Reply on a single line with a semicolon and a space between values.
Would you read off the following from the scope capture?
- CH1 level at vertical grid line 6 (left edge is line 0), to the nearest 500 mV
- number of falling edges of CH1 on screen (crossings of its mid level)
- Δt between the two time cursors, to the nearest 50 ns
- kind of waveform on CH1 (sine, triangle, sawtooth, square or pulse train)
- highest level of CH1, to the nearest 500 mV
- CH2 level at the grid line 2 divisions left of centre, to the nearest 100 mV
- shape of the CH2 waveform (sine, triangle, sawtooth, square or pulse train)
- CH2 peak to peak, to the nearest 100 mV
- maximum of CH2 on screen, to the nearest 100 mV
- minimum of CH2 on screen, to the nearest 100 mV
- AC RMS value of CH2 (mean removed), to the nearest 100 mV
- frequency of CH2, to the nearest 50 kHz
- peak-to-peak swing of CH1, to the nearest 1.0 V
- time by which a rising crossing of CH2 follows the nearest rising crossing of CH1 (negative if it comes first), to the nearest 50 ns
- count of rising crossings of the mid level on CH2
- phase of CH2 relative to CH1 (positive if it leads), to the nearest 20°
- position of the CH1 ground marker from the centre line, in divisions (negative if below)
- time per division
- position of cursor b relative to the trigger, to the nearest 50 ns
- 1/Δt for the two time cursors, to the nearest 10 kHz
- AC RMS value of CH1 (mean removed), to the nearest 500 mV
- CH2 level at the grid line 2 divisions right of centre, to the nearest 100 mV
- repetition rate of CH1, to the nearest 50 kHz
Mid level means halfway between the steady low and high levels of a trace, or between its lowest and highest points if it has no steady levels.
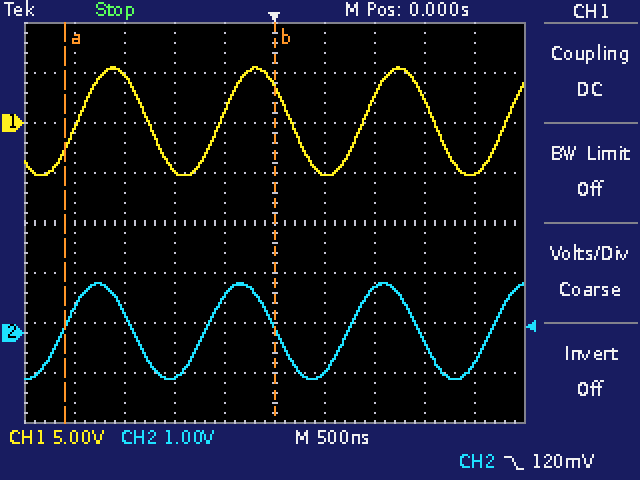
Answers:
-5.0 V; 3; 2.10 µs; sine; 5.5 V; -900 mV; sine; 1.9 V; 1.0 V; -900 mV; 700 mV; 700 kHz; 11.0 V; -150 ns; 4; +40°; +2.0 div; 500 ns; 0 ns; 480 kHz; 4.0 V; 900 mV; 700 kHz
